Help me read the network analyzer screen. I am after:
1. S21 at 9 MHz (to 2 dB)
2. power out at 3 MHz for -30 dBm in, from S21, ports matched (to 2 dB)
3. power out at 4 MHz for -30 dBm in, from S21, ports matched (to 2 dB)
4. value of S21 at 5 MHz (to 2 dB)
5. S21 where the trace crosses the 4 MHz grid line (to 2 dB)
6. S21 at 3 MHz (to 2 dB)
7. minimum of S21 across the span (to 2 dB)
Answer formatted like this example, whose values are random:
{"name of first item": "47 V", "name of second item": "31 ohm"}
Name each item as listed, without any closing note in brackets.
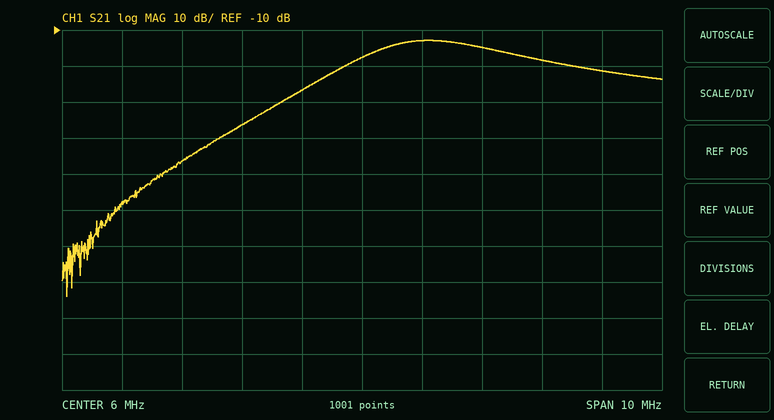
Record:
{"S21 at 9 MHz": "-18 dB", "power out at 3 MHz for -30 dBm in, from S21, ports matched": "-76 dBm", "power out at 4 MHz for -30 dBm in, from S21, ports matched": "-66 dBm", "value of S21 at 5 MHz": "-26 dB", "S21 where the trace crosses the 4 MHz grid line": "-36 dB", "S21 at 3 MHz": "-46 dB", "minimum of S21 across the span": "-84 dB"}
